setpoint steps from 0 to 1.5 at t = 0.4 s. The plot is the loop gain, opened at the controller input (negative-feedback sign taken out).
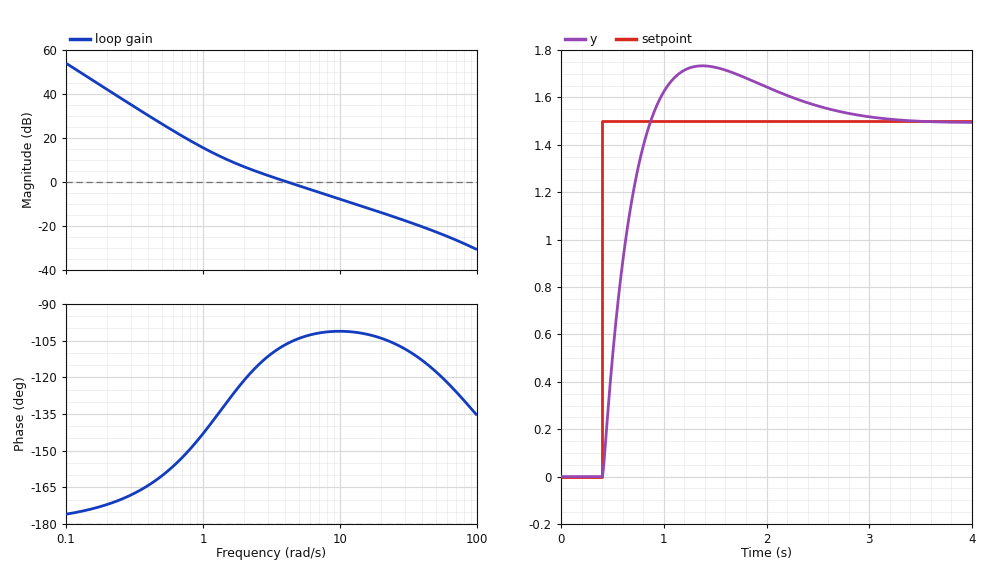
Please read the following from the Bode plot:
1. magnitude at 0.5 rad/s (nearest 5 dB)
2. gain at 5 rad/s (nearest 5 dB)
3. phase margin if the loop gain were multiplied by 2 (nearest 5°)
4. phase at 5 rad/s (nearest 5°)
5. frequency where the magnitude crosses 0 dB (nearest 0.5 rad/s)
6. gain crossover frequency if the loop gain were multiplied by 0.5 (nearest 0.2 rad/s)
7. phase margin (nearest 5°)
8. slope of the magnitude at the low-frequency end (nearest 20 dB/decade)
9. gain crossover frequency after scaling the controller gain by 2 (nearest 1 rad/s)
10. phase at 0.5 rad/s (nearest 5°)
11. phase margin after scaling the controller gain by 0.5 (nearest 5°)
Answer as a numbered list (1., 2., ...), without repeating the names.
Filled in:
1. 25 dB
2. 0 dB
3. 80°
4. -105°
5. 4.0 rad/s
6. 2.2 rad/s
7. 75°
8. -40 dB/decade
9. 8 rad/s
10. -160°
11. 60°
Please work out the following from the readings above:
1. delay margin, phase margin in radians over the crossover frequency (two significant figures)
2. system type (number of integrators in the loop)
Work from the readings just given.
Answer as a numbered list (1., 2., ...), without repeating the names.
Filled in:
1. 0.33 s
2. 2
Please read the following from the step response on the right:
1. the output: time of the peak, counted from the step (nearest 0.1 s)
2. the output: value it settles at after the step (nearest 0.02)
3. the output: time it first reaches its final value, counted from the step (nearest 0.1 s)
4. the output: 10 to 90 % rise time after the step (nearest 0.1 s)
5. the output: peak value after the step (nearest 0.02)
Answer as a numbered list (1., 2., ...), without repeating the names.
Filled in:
1. 1.0 s
2. 1.50
3. 0.5 s
4. 0.3 s
5. 1.74
